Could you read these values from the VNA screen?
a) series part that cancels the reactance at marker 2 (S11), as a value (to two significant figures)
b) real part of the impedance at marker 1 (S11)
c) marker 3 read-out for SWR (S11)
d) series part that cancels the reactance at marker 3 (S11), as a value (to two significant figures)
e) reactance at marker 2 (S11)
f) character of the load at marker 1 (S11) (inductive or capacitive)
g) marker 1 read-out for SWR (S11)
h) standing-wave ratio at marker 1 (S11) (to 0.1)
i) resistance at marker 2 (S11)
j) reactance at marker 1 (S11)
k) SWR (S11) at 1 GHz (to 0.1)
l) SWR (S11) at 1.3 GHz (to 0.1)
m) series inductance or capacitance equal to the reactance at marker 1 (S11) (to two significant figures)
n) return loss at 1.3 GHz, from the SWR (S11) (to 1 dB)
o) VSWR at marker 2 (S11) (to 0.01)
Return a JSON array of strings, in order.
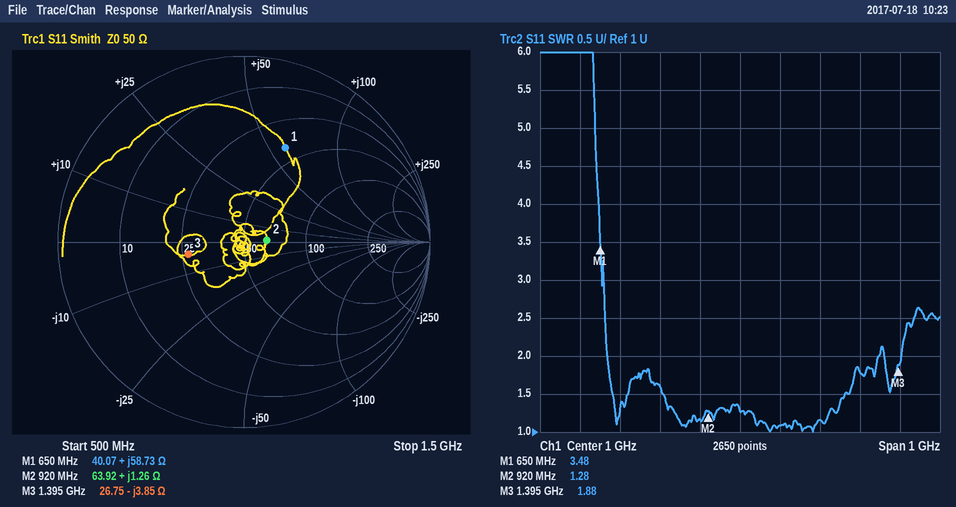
["140 pF", "40.07 Ω", "1.88", "440 pH", "+1.26 Ω", "inductive", "3.48", "3.5", "63.92 Ω", "+58.73 Ω", "1.3", "1.8", "14 nH", "11 dB", "1.28"]
